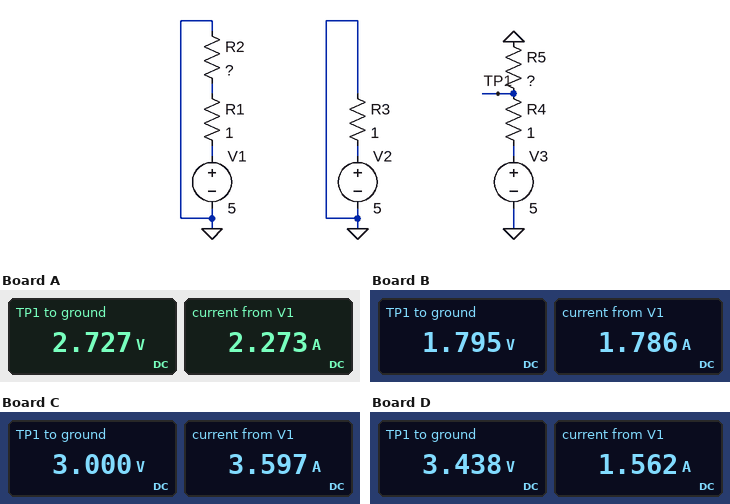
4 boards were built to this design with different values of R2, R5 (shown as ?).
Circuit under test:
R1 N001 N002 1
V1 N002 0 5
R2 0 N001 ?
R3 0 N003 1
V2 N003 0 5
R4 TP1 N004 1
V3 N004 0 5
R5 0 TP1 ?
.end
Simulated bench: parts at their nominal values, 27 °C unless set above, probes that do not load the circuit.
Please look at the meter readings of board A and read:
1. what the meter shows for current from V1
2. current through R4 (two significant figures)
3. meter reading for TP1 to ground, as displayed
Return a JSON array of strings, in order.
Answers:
["2.273 A", "2.3 A", "2.727 V"]
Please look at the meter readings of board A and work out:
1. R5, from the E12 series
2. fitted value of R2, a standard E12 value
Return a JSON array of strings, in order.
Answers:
["1.2 Ω", "1.2 Ω"]
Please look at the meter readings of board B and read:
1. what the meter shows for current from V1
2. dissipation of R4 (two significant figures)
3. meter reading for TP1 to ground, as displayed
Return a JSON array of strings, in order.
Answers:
["1.786 A", "10 W", "1.795 V"]
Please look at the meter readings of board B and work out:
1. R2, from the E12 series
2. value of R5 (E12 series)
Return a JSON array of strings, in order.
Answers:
["1.8 Ω", "0.56 Ω"]
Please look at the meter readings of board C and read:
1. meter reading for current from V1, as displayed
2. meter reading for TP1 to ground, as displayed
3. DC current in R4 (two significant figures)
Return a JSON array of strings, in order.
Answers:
["3.597 A", "3.000 V", "2.0 A"]
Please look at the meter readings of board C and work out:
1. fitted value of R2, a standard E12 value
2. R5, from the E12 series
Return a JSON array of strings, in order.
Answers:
["0.39 Ω", "1.5 Ω"]
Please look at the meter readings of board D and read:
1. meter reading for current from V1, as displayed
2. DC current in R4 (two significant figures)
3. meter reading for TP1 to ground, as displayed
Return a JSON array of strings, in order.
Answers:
["1.562 A", "1.6 A", "3.438 V"]
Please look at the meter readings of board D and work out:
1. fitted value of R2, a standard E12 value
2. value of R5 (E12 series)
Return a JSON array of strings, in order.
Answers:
["2.2 Ω", "2.2 Ω"]
